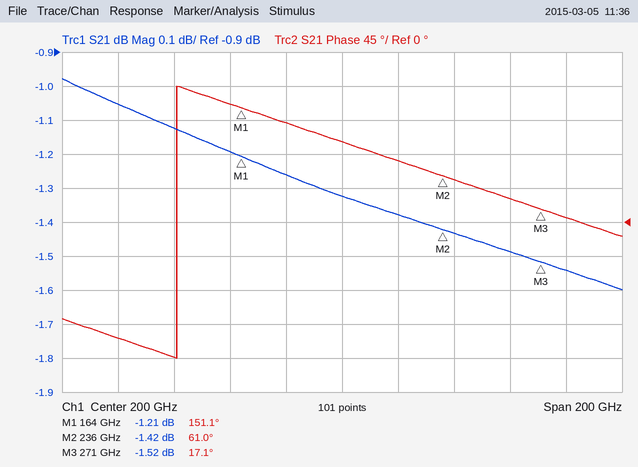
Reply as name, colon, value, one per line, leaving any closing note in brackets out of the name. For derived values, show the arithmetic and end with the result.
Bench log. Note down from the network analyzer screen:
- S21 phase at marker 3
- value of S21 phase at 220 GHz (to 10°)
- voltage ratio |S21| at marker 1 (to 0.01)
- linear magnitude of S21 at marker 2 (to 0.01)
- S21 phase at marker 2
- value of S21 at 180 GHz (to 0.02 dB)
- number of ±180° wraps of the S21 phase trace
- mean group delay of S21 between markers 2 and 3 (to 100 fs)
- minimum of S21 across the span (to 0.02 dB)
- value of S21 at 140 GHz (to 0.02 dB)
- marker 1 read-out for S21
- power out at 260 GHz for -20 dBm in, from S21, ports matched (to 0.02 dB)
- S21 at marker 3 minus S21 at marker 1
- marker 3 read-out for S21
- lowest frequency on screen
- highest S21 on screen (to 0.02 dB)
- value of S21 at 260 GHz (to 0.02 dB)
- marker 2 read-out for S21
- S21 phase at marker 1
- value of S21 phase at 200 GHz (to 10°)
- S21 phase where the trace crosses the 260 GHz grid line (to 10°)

S21 phase at marker 3: 17.1°
value of S21 phase at 220 GHz: 80°
voltage ratio |S21| at marker 1: 10^(-1.21/20) ≈ 0.87
linear magnitude of S21 at marker 2: 10^(-1.42/20) ≈ 0.85
S21 phase at marker 2: 61.0°
value of S21 at 180 GHz: -1.26 dB
number of ±180° wraps of the S21 phase trace: 1
mean group delay of S21 between markers 2 and 3: −(17.1° − (61°))/(360° × 35 GHz) ≈ 3.5 ps
minimum of S21 across the span: -1.60 dB
value of S21 at 140 GHz: -1.12 dB
marker 1 read-out for S21: -1.21 dB
power out at 260 GHz for -20 dBm in, from S21, ports matched: -20 dBm + (-1.48 dB) = -21.48 dBm
S21 at marker 3 minus S21 at marker 1: -1.52 − (-1.21) = -0.31 dB
marker 3 read-out for S21: -1.52 dB
lowest frequency on screen: 100 GHz
highest S21 on screen: -0.98 dB
value of S21 at 260 GHz: -1.48 dB
marker 2 read-out for S21: -1.42 dB
S21 phase at marker 1: 151.1°
value of S21 phase at 200 GHz: 110°
S21 phase where the trace crosses the 260 GHz grid line: 30°
